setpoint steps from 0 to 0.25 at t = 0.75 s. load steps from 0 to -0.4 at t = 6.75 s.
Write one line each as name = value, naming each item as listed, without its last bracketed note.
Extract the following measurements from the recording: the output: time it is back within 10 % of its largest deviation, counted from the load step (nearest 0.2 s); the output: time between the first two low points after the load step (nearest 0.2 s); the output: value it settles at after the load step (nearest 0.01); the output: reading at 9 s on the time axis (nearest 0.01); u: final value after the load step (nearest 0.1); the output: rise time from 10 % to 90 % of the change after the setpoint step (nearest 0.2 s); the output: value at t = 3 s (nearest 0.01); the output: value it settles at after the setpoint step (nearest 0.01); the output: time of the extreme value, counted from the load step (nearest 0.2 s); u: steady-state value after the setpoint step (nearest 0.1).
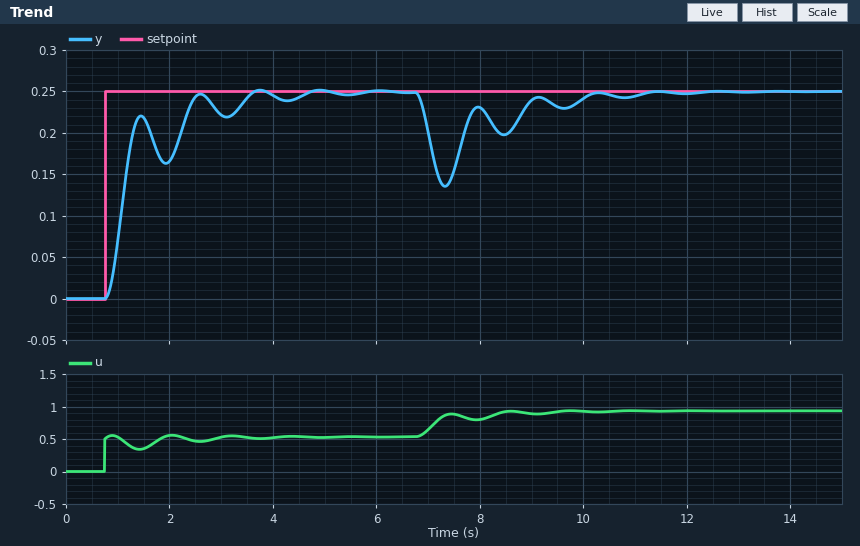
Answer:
the output: time it is back within 10 % of its largest deviation, counted from the load step = 3.2 s
the output: time between the first two low points after the load step = 1.2 s
the output: value it settles at after the load step = 0.25
the output: reading at 9 s on the time axis = 0.24
u: final value after the load step = 0.9
the output: rise time from 10 % to 90 % of the change after the setpoint step = 1.4 s
the output: value at t = 3 s = 0.22
the output: value it settles at after the setpoint step = 0.25
the output: time of the extreme value, counted from the load step = 0.6 s
u: steady-state value after the setpoint step = 0.5
